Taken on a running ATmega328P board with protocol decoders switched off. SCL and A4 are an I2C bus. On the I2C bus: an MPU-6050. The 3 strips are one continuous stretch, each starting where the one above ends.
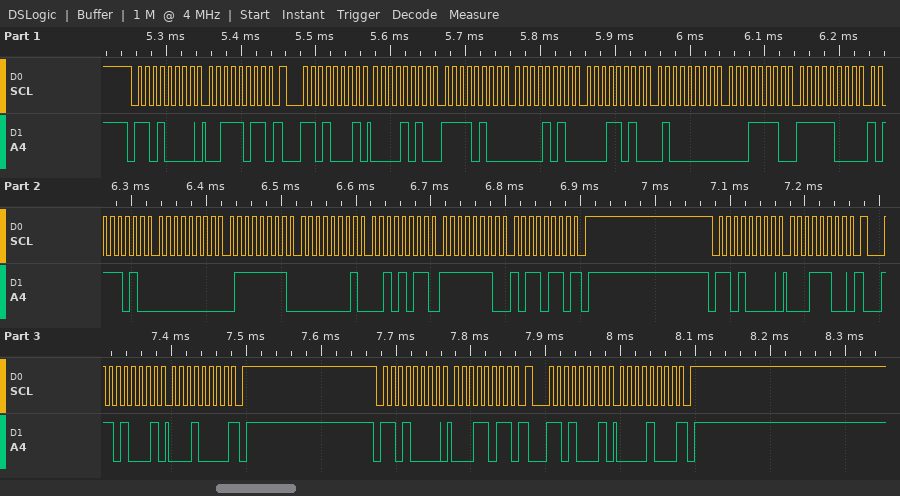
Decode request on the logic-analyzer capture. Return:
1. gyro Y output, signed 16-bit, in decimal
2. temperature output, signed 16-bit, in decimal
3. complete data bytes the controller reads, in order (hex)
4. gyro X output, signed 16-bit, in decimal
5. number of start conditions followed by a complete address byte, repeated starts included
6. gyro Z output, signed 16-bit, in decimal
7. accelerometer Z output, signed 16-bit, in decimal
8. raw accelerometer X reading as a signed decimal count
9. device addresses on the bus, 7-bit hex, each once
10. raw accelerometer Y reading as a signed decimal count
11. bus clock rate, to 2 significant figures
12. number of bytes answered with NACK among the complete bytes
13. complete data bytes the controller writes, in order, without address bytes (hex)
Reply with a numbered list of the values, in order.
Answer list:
1. 299
2. -1862
3. 0A F4 0A 1A 40 1E F8 BA 00 7F 01 2B FE B6 10 08
4. 127
5. 6
6. -330
7. 16414
8. 2804
9. 0x68
10. 2586
11. 100 kHz
12. 3
13. 3B 1C 1B
